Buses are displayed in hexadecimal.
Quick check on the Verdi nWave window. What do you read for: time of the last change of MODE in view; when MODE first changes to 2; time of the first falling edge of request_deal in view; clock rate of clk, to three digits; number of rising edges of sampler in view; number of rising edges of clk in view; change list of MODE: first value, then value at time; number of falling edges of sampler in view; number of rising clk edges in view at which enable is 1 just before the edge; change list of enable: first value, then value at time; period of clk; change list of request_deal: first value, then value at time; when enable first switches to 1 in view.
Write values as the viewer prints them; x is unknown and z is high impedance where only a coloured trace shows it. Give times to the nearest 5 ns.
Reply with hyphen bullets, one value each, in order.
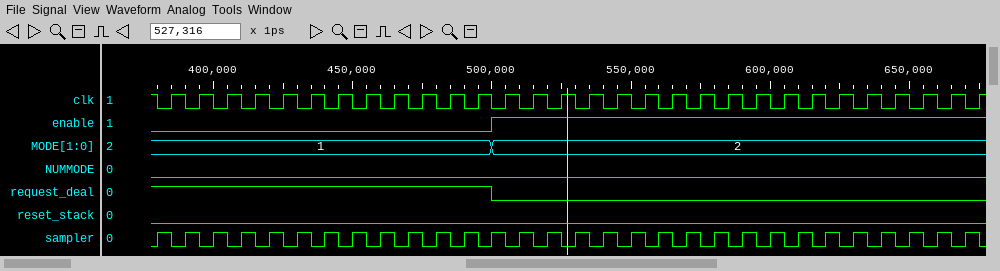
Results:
- 500 ns
- 500 ns
- 500 ns
- 100 MHz
- 30
- 30
- 1, 2 at 500 ns
- 30
- 18
- 0, 1 at 500 ns
- 10 ns
- 1, 0 at 500 ns
- 500 ns
